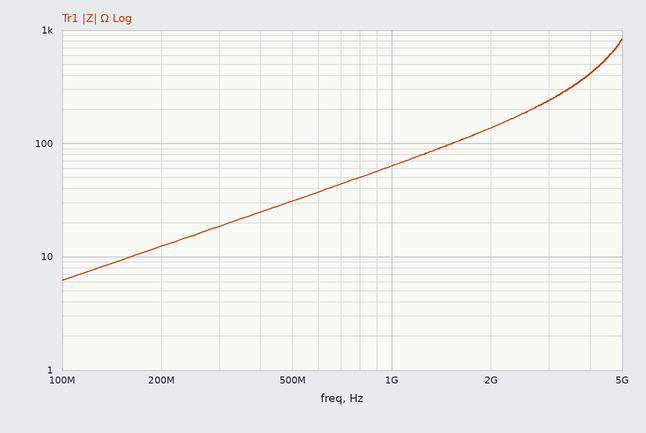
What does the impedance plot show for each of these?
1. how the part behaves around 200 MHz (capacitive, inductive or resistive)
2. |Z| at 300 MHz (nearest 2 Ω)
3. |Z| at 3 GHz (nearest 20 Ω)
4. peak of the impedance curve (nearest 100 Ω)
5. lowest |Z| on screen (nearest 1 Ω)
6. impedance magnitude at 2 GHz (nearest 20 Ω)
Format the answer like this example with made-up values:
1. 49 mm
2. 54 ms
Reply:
1. inductive
2. 18 Ω
3. 240 Ω
4. 800 Ω
5. 6 Ω
6. 140 Ω
